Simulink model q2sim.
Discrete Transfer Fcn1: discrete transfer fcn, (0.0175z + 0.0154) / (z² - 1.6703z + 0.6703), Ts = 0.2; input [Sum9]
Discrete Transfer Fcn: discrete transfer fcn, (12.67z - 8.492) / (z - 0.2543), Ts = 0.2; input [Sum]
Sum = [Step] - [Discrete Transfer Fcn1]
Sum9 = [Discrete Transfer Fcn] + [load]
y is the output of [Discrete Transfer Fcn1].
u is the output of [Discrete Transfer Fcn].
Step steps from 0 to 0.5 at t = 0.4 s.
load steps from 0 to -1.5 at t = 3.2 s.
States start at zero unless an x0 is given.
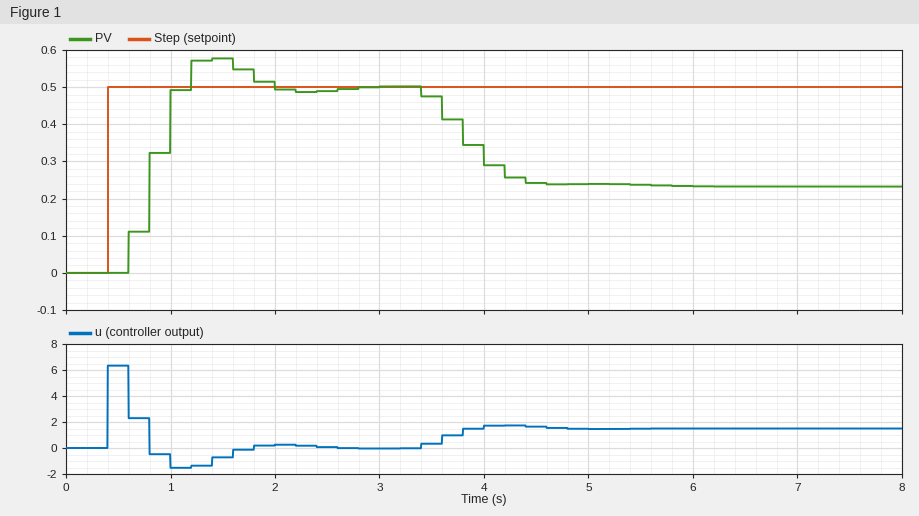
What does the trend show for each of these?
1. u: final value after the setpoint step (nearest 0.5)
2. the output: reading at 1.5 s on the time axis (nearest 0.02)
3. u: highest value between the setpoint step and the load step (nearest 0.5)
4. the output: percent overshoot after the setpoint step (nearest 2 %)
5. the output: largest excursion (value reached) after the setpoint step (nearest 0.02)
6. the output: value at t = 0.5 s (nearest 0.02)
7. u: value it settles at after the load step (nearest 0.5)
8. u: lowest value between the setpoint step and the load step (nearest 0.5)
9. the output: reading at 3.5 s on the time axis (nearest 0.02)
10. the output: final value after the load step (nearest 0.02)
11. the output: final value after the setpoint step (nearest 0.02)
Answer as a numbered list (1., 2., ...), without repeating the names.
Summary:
1. 0.0
2. 0.58
3. 6.5
4. 16 %
5. 0.58
6. 0.00
7. 1.5
8. -1.5
9. 0.48
10. 0.24
11. 0.50
